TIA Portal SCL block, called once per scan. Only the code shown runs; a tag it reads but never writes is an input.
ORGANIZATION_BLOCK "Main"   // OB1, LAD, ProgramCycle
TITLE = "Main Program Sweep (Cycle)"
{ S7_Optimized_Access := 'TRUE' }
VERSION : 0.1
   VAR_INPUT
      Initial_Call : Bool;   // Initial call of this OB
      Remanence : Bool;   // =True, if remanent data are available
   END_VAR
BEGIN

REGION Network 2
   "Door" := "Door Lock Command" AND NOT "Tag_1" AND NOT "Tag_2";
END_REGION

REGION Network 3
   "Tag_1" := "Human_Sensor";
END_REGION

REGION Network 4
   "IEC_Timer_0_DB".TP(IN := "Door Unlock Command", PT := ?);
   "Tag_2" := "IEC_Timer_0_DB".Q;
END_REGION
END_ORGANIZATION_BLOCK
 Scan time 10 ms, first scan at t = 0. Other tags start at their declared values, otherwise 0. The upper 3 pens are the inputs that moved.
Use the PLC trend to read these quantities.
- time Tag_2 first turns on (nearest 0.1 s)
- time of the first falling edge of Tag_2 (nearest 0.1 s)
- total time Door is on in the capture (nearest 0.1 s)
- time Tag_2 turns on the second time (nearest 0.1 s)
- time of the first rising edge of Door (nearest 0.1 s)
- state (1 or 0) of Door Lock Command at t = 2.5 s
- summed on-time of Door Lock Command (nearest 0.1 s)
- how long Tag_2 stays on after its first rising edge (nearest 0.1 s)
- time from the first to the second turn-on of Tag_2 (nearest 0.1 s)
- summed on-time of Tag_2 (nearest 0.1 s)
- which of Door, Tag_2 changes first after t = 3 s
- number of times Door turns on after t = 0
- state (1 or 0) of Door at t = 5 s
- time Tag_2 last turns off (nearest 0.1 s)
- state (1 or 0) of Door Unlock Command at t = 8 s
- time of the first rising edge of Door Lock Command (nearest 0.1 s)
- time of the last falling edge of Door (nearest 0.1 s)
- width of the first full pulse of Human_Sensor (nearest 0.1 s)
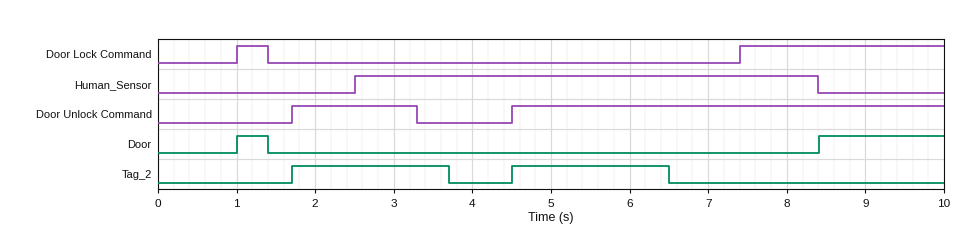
1.7 s
3.7 s
2.0 s
4.5 s
1.0 s
0
3.0 s
2.0 s
2.8 s
4.0 s
Tag_2
2
0
6.5 s
1
1.0 s
1.4 s
5.9 s
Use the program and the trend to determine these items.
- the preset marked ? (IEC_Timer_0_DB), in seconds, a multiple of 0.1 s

2.0 s
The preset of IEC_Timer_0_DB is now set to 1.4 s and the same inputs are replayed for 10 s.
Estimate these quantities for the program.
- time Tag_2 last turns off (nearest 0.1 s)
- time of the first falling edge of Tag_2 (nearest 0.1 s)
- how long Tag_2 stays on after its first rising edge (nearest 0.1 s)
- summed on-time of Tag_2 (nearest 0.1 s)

5.9 s
3.1 s
1.4 s
2.8 s
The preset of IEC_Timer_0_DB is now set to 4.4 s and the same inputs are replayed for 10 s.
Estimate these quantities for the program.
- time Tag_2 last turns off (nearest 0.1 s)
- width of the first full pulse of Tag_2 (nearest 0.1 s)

6.1 s
4.4 s
